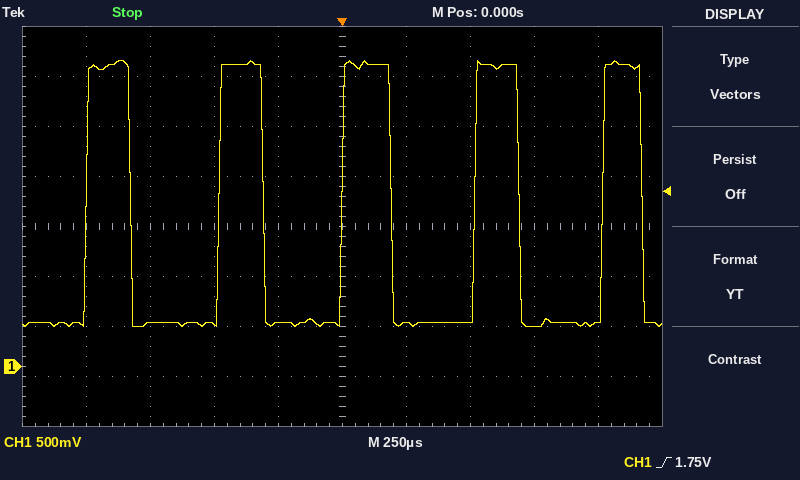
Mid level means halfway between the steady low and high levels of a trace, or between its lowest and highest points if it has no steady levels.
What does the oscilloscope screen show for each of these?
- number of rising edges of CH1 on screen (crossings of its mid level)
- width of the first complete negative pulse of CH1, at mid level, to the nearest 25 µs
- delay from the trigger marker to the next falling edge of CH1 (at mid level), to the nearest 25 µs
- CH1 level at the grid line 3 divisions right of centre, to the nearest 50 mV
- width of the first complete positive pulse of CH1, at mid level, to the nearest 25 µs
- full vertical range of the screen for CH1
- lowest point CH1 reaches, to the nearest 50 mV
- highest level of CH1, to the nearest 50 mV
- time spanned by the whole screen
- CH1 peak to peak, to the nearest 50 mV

5
350 µs
200 µs
400 mV
175 µs
4 V
400 mV
3.05 V
2.5 ms
2.65 V
